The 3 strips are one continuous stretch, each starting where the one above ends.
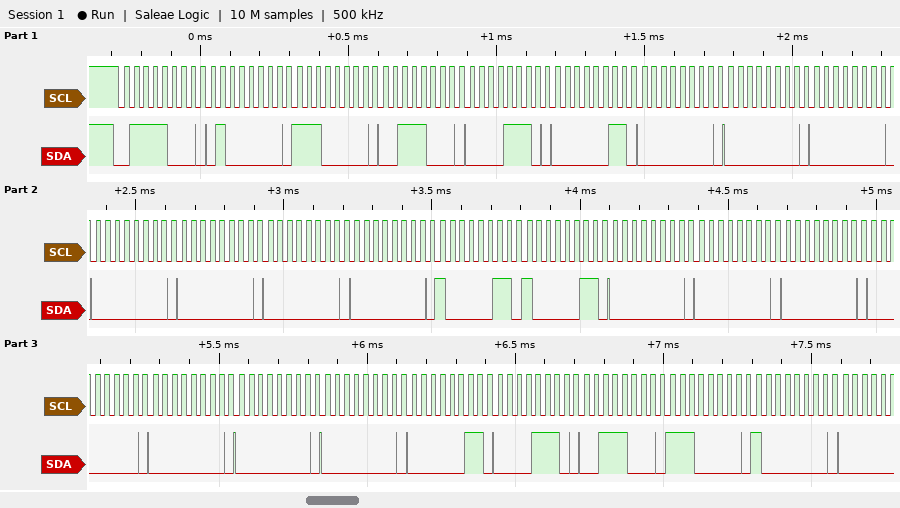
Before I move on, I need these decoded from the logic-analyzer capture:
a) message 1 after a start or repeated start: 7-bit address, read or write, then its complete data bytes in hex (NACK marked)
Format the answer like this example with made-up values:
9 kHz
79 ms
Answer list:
0x3C write: 40 E0 38 0E 03 00 00 00 00 00 00 00 83 83 00 00 00 00 00 00 00 03 0E 38 E0 80
